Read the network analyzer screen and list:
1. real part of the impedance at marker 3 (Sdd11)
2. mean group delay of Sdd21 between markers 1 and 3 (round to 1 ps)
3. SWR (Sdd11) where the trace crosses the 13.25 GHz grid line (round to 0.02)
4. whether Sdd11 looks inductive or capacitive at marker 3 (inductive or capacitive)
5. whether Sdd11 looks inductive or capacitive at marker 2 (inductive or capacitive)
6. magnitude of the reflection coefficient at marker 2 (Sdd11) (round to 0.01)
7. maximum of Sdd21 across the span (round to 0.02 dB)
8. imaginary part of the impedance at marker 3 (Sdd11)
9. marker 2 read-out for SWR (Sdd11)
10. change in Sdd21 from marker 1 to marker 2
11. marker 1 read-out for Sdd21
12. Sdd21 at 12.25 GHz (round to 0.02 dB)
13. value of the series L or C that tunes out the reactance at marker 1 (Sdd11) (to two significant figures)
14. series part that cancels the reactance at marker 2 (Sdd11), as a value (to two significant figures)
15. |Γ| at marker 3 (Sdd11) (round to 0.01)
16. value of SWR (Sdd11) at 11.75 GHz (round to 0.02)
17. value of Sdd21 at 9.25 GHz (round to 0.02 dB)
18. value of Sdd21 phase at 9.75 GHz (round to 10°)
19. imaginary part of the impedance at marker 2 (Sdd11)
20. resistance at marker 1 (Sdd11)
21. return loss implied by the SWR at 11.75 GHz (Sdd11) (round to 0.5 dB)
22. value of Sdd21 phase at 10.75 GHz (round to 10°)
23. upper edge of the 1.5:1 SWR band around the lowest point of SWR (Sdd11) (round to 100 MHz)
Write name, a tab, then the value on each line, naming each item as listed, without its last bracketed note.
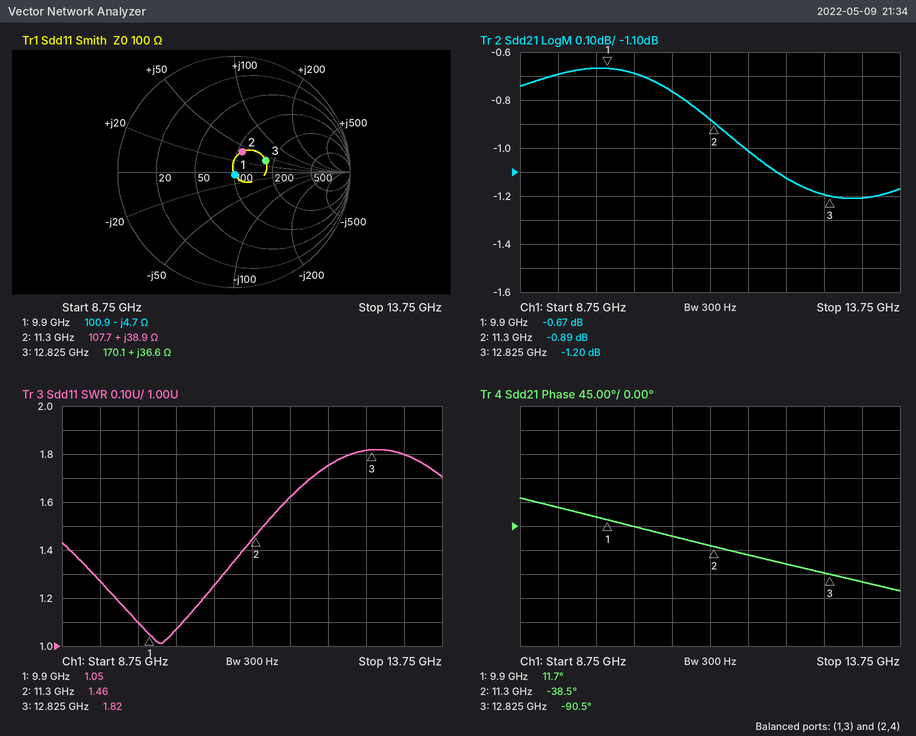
real part of the impedance at marker 3	170.1 Ω
mean group delay of Sdd21 between markers 1 and 3	97 ps
SWR (Sdd11) where the trace crosses the 13.25 GHz grid line	1.80
whether Sdd11 looks inductive or capacitive at marker 3	inductive
whether Sdd11 looks inductive or capacitive at marker 2	inductive
magnitude of the reflection coefficient at marker 2 (Sdd11)	0.19
maximum of Sdd21 across the span	-0.66 dB
imaginary part of the impedance at marker 3	+36.6 Ω
marker 2 read-out for SWR	1.46
change in Sdd21 from marker 1 to marker 2	-0.22 dB
marker 1 read-out for Sdd21	-0.67 dB
Sdd21 at 12.25 GHz	-1.12 dB
value of the series L or C that tunes out the reactance at marker 1 (Sdd11)	76 pH
series part that cancels the reactance at marker 2 (Sdd11), as a value	360 fF
|Γ| at marker 3 (Sdd11)	0.29
value of SWR (Sdd11) at 11.75 GHz	1.62
value of Sdd21 at 9.25 GHz	-0.70 dB
value of Sdd21 phase at 9.75 GHz	20°
imaginary part of the impedance at marker 2	+38.9 Ω
resistance at marker 1	100.9 Ω
return loss implied by the SWR at 11.75 GHz (Sdd11)	12.5 dB
value of Sdd21 phase at 10.75 GHz	-20°
upper edge of the 1.5:1 SWR band around the lowest point of SWR (Sdd11)	11.4 GHz
